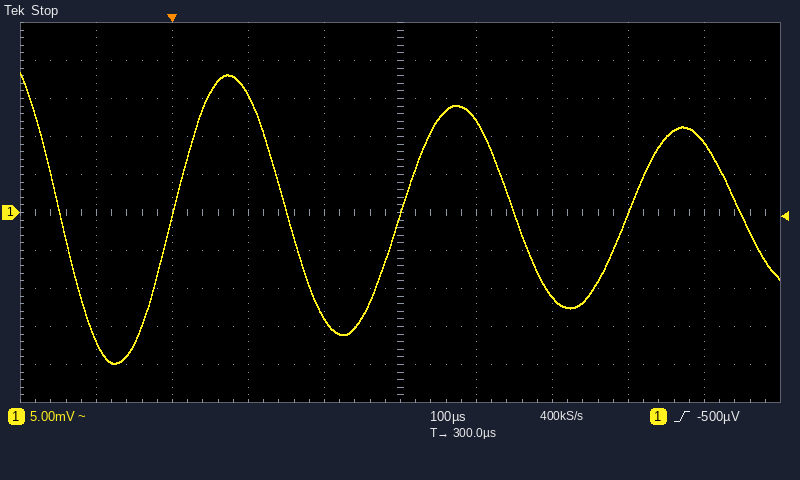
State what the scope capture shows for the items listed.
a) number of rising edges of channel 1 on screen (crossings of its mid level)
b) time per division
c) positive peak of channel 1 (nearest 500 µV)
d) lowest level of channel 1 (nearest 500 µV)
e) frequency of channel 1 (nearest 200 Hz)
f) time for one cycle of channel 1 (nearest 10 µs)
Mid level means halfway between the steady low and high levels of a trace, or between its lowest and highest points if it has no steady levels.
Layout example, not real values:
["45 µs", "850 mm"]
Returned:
["3", "100 µs", "18.5 mV", "-20.0 mV", "3.4 kHz", "300 µs"]
